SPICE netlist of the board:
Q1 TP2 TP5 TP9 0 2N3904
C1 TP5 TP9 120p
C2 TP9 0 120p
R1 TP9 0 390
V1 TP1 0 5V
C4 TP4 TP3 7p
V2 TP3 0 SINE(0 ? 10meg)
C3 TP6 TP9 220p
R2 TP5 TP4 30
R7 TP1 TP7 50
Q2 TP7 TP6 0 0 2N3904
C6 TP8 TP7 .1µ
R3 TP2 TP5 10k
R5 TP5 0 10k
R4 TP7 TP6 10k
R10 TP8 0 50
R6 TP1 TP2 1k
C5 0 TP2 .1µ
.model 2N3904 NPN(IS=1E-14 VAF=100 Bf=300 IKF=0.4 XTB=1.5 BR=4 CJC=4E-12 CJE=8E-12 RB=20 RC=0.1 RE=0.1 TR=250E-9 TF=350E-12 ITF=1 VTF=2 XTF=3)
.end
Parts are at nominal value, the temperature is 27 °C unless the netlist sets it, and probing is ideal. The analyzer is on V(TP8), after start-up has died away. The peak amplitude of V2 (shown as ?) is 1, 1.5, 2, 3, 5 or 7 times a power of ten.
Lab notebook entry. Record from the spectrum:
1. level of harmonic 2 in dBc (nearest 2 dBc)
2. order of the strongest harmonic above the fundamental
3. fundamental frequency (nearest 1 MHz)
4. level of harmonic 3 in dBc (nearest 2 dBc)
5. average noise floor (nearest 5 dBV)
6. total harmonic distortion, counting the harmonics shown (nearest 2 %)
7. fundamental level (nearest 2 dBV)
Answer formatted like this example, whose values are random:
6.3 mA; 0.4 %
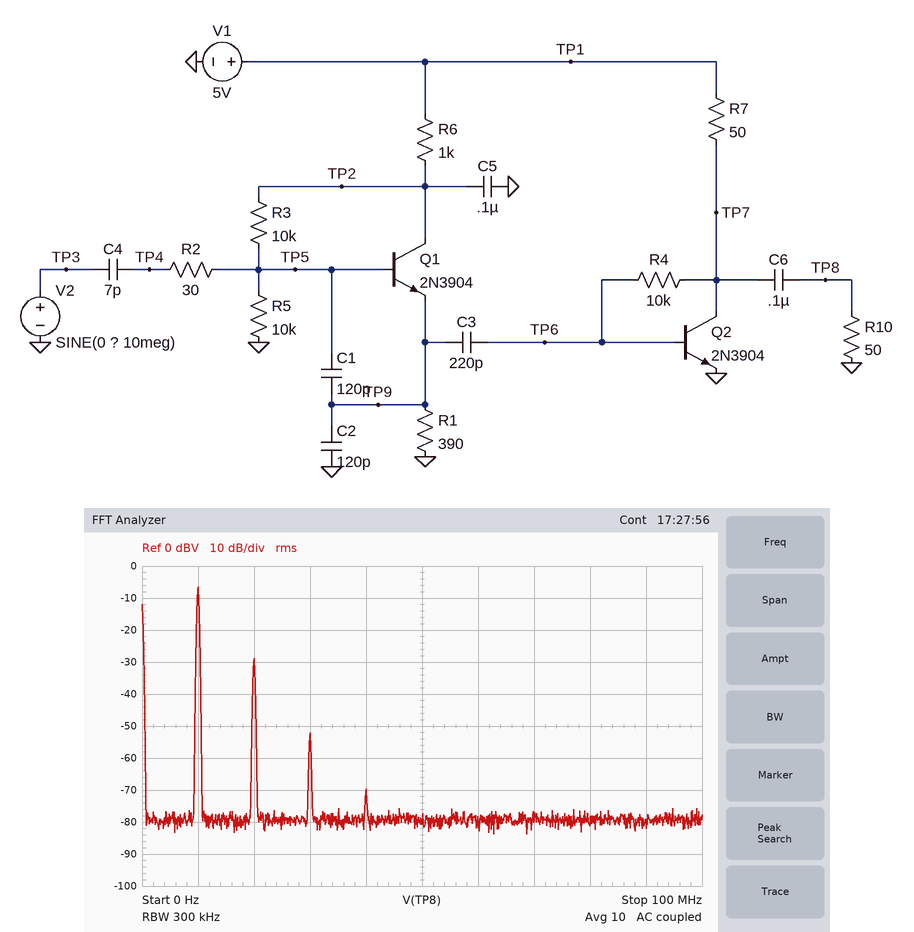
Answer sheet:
-22 dBc; 2; 10 MHz; -46 dBc; -80 dBV; 8 %; -6 dBV
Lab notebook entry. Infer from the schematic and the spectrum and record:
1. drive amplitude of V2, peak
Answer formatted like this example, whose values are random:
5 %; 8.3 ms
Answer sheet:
500 mV
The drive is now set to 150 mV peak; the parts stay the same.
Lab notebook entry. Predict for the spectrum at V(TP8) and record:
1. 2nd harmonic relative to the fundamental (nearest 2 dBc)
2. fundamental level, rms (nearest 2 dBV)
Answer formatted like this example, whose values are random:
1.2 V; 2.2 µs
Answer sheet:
-32 dBc; -16 dBV
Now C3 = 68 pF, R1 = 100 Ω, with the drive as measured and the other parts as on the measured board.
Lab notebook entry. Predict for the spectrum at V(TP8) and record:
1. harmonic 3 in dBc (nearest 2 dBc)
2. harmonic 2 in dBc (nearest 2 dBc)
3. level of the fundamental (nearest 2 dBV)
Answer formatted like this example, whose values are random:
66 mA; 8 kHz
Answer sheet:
-56 dBc; -24 dBc; -12 dBV
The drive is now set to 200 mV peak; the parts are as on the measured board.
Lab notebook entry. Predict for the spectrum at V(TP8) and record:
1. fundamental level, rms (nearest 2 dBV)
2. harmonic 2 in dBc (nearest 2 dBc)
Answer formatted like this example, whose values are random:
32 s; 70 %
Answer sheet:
-14 dBV; -30 dBc
